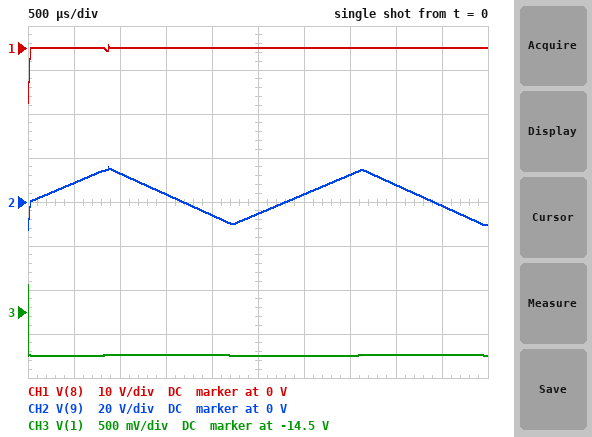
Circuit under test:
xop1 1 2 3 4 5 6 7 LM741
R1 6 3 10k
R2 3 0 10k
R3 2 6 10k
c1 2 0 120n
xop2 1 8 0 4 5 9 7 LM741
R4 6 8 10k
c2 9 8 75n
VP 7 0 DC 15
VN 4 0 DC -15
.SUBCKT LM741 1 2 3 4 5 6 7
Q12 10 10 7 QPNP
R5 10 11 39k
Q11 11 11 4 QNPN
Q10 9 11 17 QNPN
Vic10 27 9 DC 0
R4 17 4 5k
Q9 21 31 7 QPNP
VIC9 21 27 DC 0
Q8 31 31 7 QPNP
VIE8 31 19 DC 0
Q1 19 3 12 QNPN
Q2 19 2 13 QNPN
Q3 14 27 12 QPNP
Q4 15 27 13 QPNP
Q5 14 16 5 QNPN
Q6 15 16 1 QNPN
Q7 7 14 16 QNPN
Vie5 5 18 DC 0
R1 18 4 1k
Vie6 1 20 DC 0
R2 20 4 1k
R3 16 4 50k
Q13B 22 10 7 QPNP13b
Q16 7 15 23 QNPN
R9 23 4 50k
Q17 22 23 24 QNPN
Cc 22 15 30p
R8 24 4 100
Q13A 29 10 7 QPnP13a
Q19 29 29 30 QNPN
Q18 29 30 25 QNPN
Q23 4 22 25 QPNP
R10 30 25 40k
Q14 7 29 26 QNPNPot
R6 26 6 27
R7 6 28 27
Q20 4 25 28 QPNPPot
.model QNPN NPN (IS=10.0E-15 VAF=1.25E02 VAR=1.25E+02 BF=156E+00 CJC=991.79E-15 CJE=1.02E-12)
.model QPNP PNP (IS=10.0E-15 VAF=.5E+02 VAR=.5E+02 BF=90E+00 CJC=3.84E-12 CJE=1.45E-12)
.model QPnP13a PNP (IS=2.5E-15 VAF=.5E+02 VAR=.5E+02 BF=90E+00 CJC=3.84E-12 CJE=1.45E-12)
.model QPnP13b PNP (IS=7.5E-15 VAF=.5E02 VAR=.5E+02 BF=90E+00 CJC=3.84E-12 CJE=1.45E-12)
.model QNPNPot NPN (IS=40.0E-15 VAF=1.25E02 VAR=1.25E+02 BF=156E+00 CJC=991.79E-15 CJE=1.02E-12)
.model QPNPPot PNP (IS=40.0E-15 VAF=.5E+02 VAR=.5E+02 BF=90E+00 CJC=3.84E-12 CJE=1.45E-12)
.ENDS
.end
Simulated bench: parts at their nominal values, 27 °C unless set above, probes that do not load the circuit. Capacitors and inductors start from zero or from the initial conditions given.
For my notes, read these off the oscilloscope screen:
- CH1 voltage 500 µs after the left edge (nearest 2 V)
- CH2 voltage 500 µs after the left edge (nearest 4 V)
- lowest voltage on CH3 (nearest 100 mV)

0 V
8 V
-15.0 V
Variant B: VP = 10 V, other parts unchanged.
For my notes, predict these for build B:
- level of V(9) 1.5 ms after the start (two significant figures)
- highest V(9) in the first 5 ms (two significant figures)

6.0 V
11 V
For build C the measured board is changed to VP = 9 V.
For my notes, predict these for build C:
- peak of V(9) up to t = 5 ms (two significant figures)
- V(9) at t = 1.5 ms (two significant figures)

10 V
6.2 V
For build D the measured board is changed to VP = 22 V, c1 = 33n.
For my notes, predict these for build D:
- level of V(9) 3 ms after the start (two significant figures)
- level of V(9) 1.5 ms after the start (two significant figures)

-6.2 V
-7.4 V
